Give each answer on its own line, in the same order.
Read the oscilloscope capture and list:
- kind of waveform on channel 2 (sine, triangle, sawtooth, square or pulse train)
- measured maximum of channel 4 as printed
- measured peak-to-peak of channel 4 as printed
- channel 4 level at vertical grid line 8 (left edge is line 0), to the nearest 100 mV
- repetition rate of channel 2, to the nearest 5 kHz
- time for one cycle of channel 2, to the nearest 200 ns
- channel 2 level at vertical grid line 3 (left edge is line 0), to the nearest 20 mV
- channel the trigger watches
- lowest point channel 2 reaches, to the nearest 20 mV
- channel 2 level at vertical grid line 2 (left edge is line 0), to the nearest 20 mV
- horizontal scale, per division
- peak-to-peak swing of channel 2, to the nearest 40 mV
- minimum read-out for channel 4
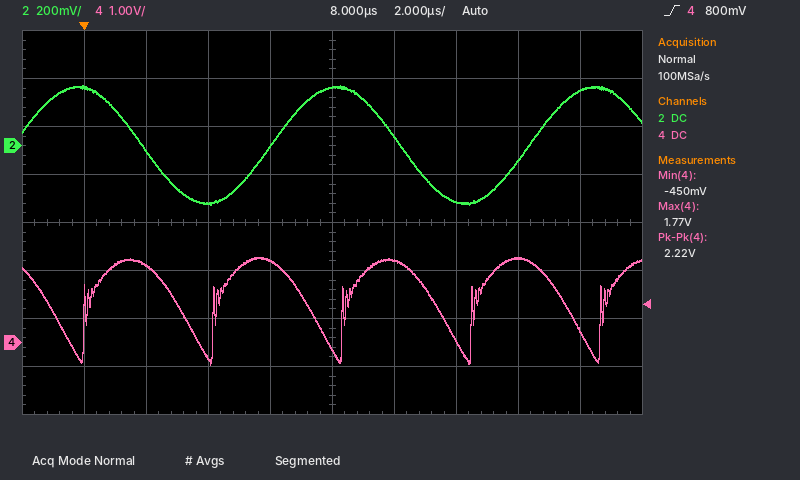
sine
1.77 V
2.22 V
1.8 V
120 kHz
8.4 µs
-240 mV
channel 4
-240 mV
-20 mV
2 µs
480 mV
-450 mV
